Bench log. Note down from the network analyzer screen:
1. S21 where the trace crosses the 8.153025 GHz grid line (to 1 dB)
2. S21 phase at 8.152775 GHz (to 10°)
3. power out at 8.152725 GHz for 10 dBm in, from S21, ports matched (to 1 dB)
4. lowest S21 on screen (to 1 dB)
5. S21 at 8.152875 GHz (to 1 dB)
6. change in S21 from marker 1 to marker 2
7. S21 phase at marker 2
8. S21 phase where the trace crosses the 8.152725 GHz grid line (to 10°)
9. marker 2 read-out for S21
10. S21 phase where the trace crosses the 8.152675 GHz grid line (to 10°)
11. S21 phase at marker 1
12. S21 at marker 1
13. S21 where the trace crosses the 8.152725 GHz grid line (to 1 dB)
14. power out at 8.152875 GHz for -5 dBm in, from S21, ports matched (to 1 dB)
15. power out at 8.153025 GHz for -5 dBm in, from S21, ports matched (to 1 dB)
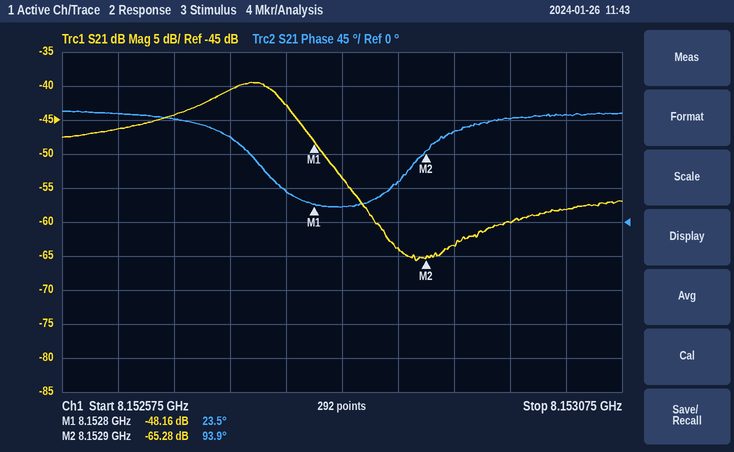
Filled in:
-58 dB
40°
-31 dBm
-66 dB
-64 dB
-17.12 dB
93.9°
110°
-65.28 dB
140°
23.5°
-48.16 dB
-41 dB
-69 dBm
-63 dBm
